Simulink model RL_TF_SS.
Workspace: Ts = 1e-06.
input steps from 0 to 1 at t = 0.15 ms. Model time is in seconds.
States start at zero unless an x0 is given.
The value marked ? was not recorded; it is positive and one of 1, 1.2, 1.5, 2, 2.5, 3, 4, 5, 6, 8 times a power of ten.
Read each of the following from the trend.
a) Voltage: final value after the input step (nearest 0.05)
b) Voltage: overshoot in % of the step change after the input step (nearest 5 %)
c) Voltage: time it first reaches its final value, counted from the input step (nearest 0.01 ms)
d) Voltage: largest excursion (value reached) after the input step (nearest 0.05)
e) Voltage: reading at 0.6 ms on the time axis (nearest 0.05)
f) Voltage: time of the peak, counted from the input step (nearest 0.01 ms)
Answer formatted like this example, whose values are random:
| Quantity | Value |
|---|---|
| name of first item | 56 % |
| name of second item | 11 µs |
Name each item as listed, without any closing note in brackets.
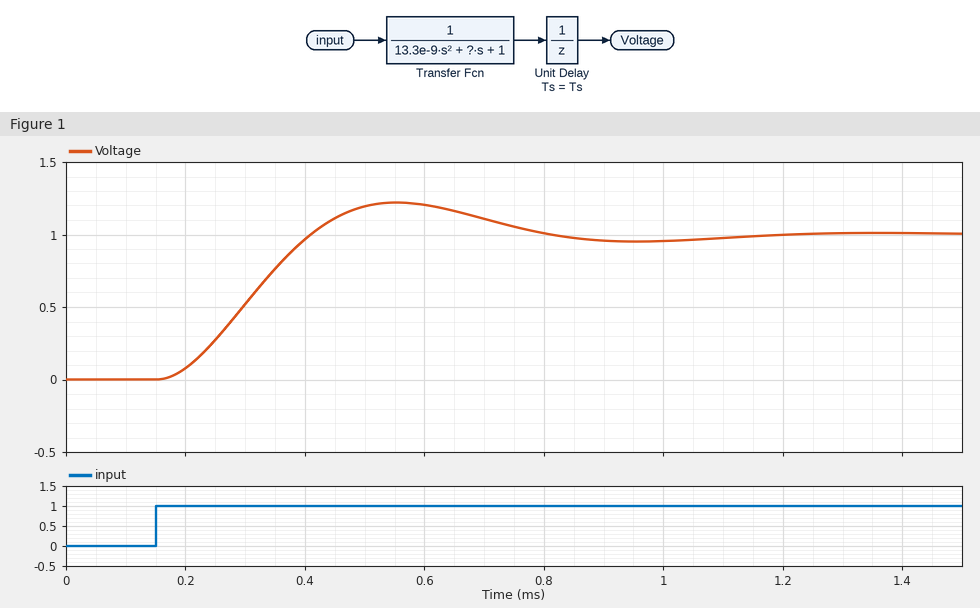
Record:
| Quantity | Value |
|---|---|
| Voltage: final value after the input step | 1.00 |
| Voltage: overshoot in % of the step change after the input step | 20 % |
| Voltage: time it first reaches its final value, counted from the input step | 0.26 ms |
| Voltage: largest excursion (value reached) after the input step | 1.20 |
| Voltage: reading at 0.6 ms on the time axis | 1.20 |
| Voltage: time of the peak, counted from the input step | 0.40 ms |
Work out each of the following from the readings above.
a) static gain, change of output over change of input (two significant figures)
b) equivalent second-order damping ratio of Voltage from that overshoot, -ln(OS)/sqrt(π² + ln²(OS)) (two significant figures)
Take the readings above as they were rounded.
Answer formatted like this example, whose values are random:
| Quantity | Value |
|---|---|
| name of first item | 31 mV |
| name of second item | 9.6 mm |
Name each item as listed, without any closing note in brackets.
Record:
| Quantity | Value |
|---|---|
| static gain, change of output over change of input | 1.0 |
| equivalent second-order damping ratio of Voltage from that overshoot, -ln(OS)/sqrt(π² + ln²(OS)) | 0.46 |
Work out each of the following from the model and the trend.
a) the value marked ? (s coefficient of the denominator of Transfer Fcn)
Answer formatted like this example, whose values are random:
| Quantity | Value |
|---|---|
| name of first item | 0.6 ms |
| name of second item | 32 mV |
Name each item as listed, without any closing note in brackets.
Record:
| Quantity | Value |
|---|---|
| the value marked ? | 0.0001 |
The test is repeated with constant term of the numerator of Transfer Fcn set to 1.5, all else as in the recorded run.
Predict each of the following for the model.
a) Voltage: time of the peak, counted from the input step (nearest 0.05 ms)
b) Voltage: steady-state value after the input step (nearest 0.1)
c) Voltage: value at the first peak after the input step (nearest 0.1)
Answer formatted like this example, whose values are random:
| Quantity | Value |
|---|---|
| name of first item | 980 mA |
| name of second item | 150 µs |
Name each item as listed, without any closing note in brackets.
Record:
| Quantity | Value |
|---|---|
| Voltage: time of the peak, counted from the input step | 0.40 ms |
| Voltage: steady-state value after the input step | 1.5 |
| Voltage: value at the first peak after the input step | 1.8 |
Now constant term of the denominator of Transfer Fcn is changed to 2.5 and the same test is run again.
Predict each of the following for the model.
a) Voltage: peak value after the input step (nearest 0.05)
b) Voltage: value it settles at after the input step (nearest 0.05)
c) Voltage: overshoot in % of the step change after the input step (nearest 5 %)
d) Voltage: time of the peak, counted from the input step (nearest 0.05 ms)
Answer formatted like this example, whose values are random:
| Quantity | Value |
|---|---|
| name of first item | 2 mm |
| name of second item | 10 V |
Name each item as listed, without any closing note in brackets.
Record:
| Quantity | Value |
|---|---|
| Voltage: peak value after the input step | 0.55 |
| Voltage: value it settles at after the input step | 0.40 |
| Voltage: overshoot in % of the step change after the input step | 40 % |
| Voltage: time of the peak, counted from the input step | 0.25 ms |
